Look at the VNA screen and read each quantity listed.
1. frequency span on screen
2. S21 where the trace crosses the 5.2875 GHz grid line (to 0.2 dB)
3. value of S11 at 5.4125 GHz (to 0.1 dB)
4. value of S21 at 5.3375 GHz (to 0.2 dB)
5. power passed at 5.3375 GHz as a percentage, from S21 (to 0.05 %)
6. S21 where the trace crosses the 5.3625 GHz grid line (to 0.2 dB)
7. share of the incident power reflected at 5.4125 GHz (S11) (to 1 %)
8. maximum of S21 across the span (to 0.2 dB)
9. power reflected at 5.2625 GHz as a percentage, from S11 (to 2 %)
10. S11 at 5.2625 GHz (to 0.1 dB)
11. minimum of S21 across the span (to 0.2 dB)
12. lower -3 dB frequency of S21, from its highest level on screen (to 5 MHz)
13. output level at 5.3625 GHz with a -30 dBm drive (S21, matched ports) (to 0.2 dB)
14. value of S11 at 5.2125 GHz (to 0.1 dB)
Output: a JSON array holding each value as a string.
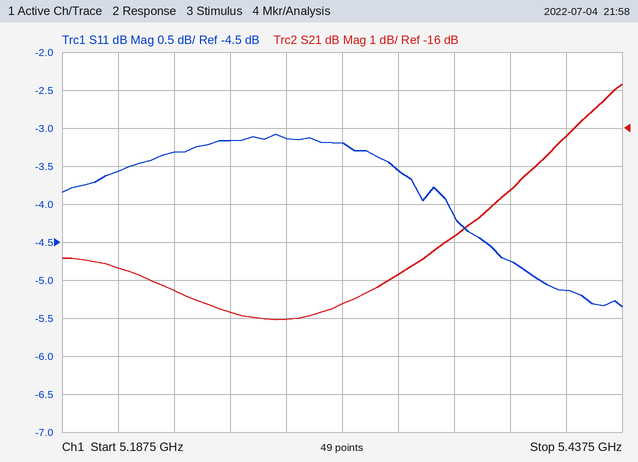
["250 MHz", "-21.0 dB", "-5.1 dB", "-19.8 dB", "1.05 %", "-18.8 dB", "31 %", "-14.8 dB", "48 %", "-3.2 dB", "-21.0 dB", "5.385 GHz", "-48.8 dBm", "-3.6 dB"]
